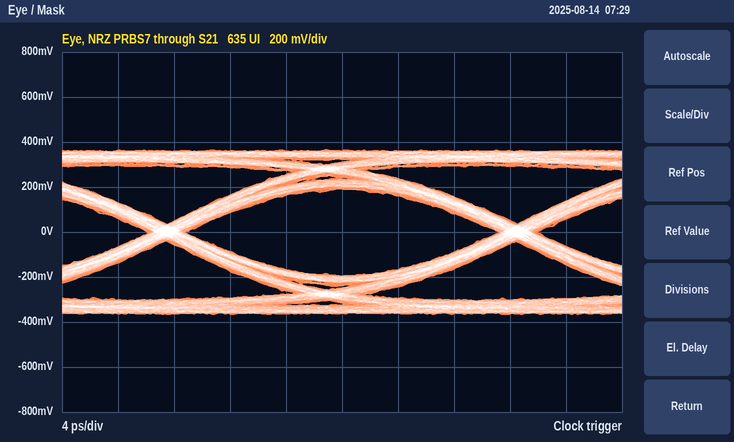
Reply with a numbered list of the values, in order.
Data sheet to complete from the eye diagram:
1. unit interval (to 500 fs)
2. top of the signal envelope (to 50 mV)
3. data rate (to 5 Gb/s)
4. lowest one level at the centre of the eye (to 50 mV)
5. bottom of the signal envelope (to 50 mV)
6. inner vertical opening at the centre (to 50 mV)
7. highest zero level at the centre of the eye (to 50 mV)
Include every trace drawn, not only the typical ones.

1. 25.0 ps
2. 350 mV
3. 40 Gb/s
4. 200 mV
5. -350 mV
6. 400 mV
7. -200 mV
